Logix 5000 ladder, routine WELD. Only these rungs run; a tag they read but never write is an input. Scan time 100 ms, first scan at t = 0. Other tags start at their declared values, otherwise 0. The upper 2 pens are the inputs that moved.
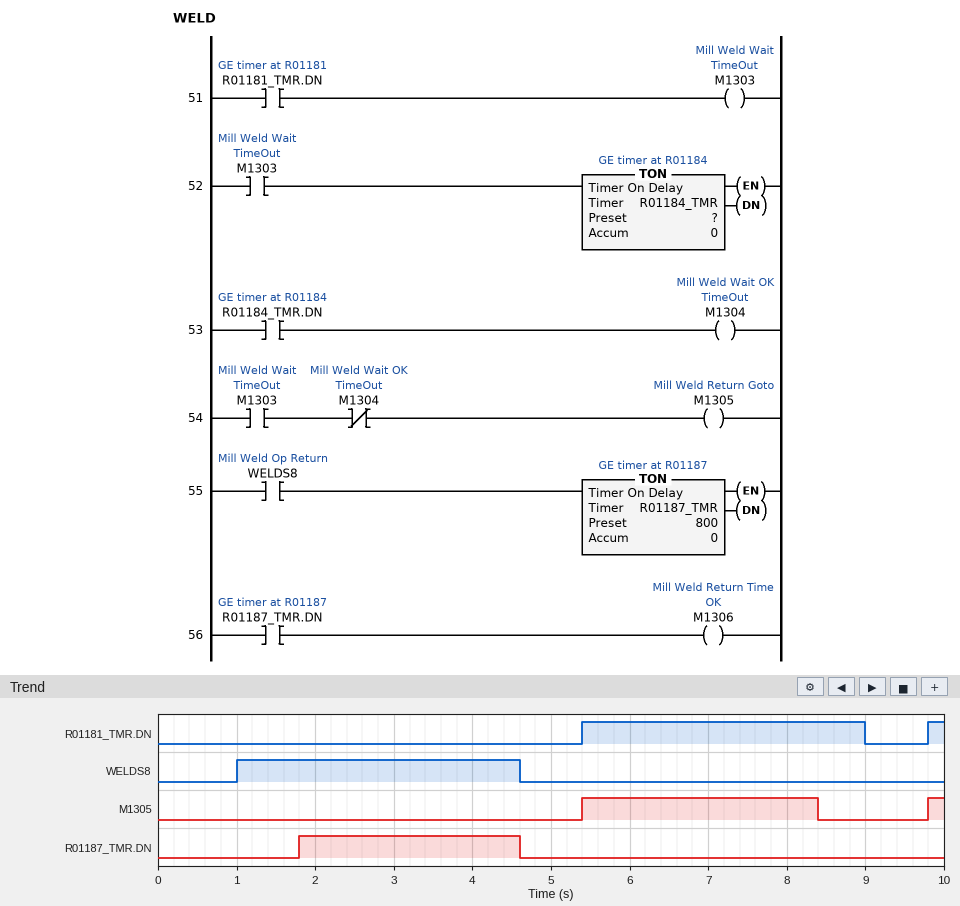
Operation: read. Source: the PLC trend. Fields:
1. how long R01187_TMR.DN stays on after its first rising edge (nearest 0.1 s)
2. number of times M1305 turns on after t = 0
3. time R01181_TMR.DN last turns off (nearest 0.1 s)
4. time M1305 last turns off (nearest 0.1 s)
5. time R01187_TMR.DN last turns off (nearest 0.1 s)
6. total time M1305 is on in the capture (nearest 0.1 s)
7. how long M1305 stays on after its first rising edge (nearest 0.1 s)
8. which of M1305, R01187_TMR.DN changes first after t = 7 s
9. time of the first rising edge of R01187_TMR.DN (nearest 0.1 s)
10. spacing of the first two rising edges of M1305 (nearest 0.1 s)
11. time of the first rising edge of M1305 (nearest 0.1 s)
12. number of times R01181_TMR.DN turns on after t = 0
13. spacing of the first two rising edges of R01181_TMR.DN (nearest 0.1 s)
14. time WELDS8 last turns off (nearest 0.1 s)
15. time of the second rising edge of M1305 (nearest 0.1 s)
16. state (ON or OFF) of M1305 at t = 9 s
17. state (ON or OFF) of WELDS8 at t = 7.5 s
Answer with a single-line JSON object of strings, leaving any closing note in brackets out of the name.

{"how long R01187_TMR.DN stays on after its first rising edge": "2.8 s", "number of times M1305 turns on after t = 0": "2", "time R01181_TMR.DN last turns off": "9.0 s", "time M1305 last turns off": "8.4 s", "time R01187_TMR.DN last turns off": "4.6 s", "total time M1305 is on in the capture": "3.2 s", "how long M1305 stays on after its first rising edge": "3.0 s", "which of M1305, R01187_TMR.DN changes first after t = 7 s": "M1305", "time of the first rising edge of R01187_TMR.DN": "1.8 s", "spacing of the first two rising edges of M1305": "4.4 s", "time of the first rising edge of M1305": "5.4 s", "number of times R01181_TMR.DN turns on after t = 0": "2", "spacing of the first two rising edges of R01181_TMR.DN": "4.4 s", "time WELDS8 last turns off": "4.6 s", "time of the second rising edge of M1305": "9.8 s", "state (ON or OFF) of M1305 at t = 9 s": "OFF", "state (ON or OFF) of WELDS8 at t = 7.5 s": "OFF"}
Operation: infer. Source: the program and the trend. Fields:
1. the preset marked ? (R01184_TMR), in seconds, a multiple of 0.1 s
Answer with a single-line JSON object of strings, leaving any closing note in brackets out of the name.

{"the preset marked ? (R01184_TMR), in seconds, a multiple of 0.1 s": "3.0 s"}
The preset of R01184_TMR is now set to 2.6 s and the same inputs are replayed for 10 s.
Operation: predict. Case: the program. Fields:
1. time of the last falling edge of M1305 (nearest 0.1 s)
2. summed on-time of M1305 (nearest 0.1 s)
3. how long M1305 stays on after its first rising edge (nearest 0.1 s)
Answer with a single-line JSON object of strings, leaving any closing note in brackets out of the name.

{"time of the last falling edge of M1305": "8.0 s", "summed on-time of M1305": "2.8 s", "how long M1305 stays on after its first rising edge": "2.6 s"}
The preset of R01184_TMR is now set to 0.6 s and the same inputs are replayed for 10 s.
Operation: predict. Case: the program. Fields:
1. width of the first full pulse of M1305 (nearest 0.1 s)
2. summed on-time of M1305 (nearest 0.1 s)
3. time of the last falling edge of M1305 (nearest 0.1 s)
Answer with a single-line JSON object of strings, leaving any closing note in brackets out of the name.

{"width of the first full pulse of M1305": "0.6 s", "summed on-time of M1305": "0.8 s", "time of the last falling edge of M1305": "6.0 s"}
